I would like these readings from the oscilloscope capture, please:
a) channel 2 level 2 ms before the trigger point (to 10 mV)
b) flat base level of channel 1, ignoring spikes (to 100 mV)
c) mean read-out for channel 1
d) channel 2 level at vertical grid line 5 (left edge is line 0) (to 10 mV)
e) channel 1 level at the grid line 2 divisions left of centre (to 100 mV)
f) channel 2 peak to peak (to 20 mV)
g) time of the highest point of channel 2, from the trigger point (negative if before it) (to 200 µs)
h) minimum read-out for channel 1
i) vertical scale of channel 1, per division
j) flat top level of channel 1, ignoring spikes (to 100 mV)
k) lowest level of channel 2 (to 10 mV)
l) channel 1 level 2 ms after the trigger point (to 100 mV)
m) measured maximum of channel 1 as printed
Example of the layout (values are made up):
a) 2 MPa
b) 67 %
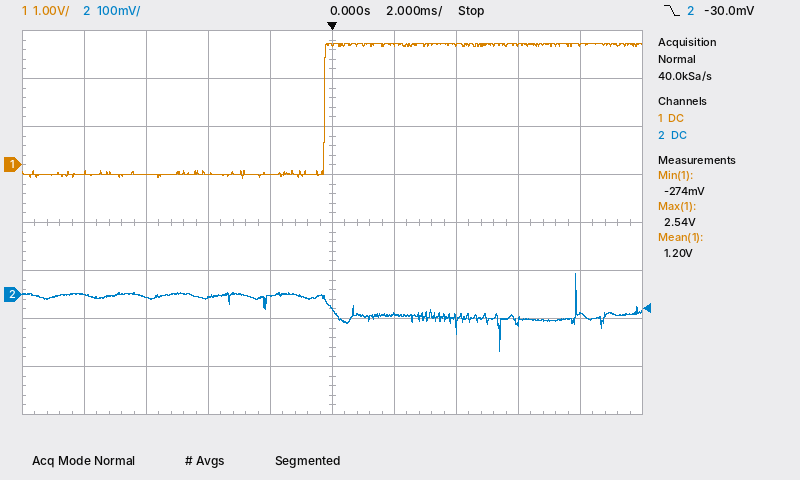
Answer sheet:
a) 0 mV
b) -200 mV
c) 1.20 V
d) -30 mV
e) -200 mV
f) 160 mV
g) +7.8 ms
h) -274 mV
i) 1 V
j) 2.5 V
k) -120 mV
l) 2.5 V
m) 2.54 V
